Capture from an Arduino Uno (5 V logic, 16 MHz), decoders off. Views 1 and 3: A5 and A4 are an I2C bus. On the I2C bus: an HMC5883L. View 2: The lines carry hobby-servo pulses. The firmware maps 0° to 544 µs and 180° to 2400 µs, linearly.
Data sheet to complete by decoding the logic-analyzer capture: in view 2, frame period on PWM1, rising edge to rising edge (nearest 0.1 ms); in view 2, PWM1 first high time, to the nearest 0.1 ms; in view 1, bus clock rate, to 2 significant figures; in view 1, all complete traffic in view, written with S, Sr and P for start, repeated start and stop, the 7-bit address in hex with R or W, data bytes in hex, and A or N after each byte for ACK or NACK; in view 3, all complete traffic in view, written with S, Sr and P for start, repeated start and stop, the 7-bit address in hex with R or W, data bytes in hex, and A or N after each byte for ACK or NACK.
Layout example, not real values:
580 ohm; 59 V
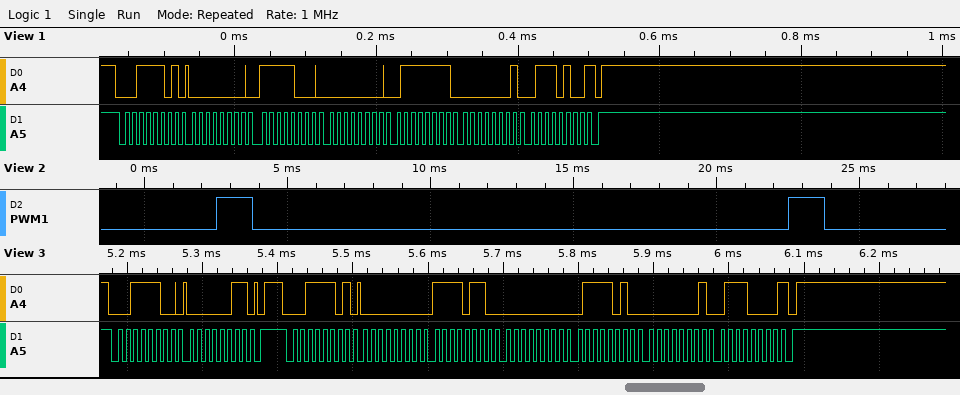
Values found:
20.0 ms; 1.3 ms; 100 kHz; S 1ER A 00 A F8 A 00 A 7F A 01 A 74 N P; S 1EW A 03 A P S 1ER A 00 A F6 A 00 A 7A A 01 A 70 N P
